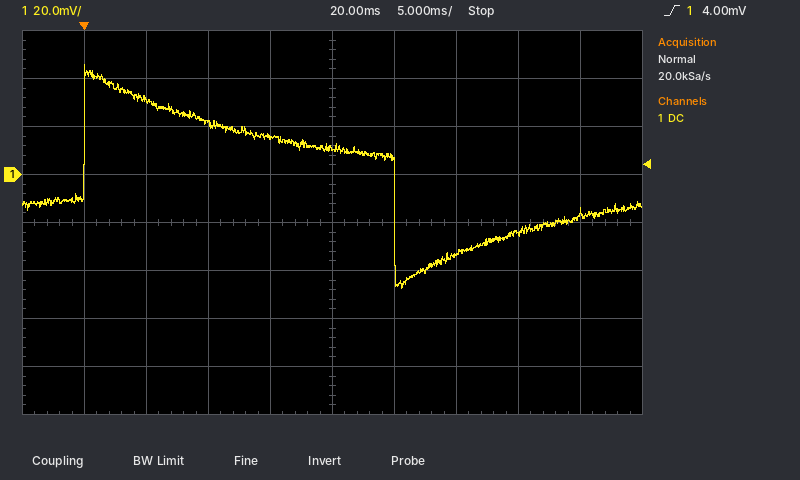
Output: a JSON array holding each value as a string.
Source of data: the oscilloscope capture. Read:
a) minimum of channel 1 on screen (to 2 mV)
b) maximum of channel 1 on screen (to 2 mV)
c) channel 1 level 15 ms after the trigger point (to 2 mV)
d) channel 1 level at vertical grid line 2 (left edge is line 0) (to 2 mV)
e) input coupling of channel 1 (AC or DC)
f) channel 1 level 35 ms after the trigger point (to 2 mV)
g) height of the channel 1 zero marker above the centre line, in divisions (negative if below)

["-48 mV", "46 mV", "16 mV", "32 mV", "DC", "-24 mV", "+1.0 div"]
